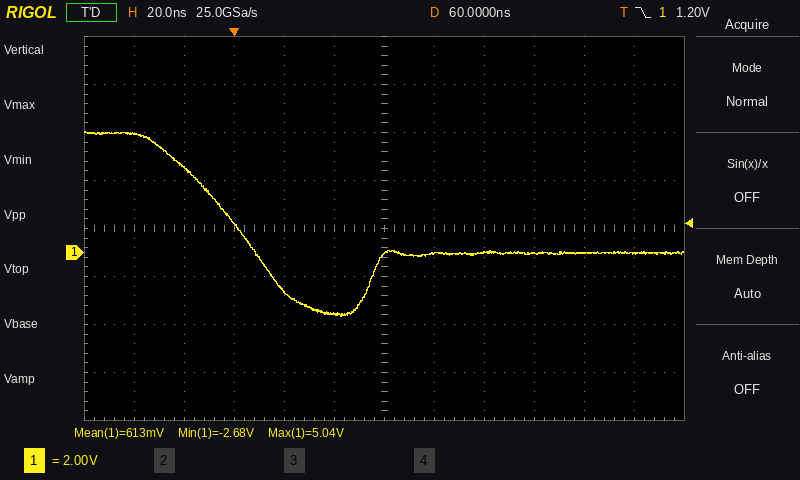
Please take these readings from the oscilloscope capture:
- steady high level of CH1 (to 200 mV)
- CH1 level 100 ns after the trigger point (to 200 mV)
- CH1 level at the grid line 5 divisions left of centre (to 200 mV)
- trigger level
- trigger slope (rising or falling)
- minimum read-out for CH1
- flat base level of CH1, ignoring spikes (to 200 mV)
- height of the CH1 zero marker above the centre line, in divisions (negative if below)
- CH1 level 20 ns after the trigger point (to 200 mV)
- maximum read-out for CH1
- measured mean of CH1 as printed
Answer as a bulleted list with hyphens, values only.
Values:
- 5.0 V
- 0.0 V
- 5.0 V
- 1.20 V
- falling
- -2.68 V
- 0.0 V
- -0.5 div
- -1.6 V
- 5.04 V
- 613 mV
